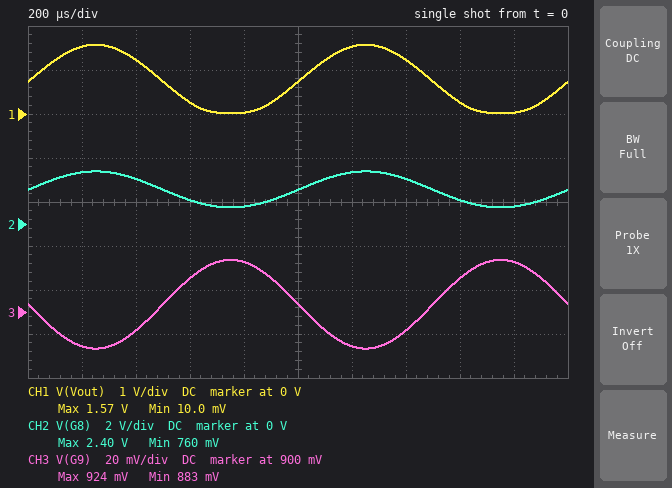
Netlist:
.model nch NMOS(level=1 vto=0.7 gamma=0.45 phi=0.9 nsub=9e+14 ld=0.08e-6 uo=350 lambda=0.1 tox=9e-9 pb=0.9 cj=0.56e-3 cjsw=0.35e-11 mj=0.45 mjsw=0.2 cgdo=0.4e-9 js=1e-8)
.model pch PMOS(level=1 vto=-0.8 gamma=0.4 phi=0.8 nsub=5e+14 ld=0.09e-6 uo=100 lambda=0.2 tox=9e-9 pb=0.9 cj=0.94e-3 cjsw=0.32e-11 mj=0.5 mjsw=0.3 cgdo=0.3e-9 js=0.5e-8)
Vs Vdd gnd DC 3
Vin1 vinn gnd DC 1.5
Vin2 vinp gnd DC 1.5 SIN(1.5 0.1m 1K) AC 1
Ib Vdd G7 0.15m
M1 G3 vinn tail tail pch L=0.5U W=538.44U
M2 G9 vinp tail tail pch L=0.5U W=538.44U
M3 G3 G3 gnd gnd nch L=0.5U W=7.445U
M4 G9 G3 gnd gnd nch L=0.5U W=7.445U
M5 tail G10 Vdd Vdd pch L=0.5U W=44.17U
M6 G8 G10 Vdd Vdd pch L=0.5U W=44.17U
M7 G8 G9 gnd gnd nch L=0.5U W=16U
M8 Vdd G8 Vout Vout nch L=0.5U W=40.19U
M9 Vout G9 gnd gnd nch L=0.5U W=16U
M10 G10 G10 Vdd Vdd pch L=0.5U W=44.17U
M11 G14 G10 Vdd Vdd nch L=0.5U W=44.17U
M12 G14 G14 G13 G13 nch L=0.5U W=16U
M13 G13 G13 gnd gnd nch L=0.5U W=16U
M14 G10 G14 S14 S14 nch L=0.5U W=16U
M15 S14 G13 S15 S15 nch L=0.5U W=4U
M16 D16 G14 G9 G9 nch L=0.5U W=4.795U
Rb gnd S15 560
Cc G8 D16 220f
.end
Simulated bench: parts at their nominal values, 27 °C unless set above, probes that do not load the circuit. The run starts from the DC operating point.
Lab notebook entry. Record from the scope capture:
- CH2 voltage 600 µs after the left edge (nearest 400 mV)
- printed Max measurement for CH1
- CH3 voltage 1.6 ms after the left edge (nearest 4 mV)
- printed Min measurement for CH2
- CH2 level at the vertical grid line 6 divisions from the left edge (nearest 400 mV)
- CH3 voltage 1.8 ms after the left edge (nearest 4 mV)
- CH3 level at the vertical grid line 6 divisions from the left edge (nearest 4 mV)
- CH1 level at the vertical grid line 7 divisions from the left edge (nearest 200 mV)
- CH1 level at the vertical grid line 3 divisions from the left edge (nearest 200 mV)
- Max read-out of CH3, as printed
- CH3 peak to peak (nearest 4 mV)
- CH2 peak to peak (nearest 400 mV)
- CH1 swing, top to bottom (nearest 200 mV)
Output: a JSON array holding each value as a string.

["1.2 V", "1.57 V", "916 mV", "760 mV", "2.4 V", "924 mV", "884 mV", "1.2 V", "200 mV", "924 mV", "40 mV", "1.6 V", "1.6 V"]
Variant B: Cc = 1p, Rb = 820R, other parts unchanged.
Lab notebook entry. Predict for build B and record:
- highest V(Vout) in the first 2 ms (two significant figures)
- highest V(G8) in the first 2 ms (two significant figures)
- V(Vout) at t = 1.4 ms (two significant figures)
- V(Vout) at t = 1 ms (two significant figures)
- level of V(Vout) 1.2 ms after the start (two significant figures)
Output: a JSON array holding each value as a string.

["1.7 V", "2.5 V", "1.3 V", "720 mV", "1.6 V"]
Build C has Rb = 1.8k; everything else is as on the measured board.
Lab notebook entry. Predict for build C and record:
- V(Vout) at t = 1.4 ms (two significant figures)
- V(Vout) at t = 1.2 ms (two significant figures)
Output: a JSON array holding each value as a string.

["1.5 V", "2.0 V"]
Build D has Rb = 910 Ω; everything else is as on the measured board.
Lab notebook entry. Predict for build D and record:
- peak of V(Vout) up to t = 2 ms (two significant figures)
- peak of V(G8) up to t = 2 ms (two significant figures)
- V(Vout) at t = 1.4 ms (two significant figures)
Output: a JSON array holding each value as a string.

["1.7 V", "2.5 V", "1.3 V"]
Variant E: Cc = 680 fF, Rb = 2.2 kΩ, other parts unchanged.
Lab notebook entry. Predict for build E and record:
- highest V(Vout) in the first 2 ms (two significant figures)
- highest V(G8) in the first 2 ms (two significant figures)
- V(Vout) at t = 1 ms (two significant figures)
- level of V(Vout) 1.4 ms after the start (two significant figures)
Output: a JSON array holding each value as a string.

["2.1 V", "2.9 V", "700 mV", "1.6 V"]
